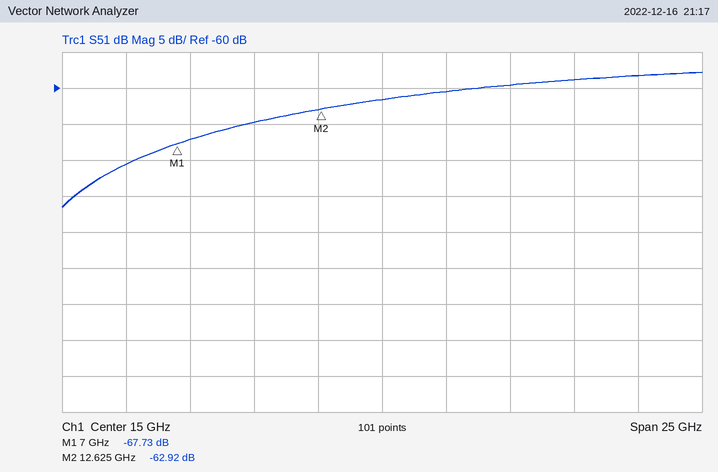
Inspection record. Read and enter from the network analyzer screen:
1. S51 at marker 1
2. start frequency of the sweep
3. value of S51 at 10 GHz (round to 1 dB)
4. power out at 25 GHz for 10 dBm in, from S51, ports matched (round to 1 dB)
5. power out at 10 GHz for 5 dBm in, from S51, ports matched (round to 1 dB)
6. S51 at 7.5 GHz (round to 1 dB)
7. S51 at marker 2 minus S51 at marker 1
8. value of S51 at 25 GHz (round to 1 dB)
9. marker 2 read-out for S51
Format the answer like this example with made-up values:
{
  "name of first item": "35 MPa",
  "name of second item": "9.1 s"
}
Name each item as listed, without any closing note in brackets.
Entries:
{
  "S51 at marker 1": "-67.73 dB",
  "start frequency of the sweep": "2.5 GHz",
  "value of S51 at 10 GHz": "-65 dB",
  "power out at 25 GHz for 10 dBm in, from S51, ports matched": "-48 dBm",
  "power out at 10 GHz for 5 dBm in, from S51, ports matched": "-60 dBm",
  "S51 at 7.5 GHz": "-67 dB",
  "S51 at marker 2 minus S51 at marker 1": "4.81 dB",
  "value of S51 at 25 GHz": "-58 dB",
  "marker 2 read-out for S51": "-62.92 dB"
}
